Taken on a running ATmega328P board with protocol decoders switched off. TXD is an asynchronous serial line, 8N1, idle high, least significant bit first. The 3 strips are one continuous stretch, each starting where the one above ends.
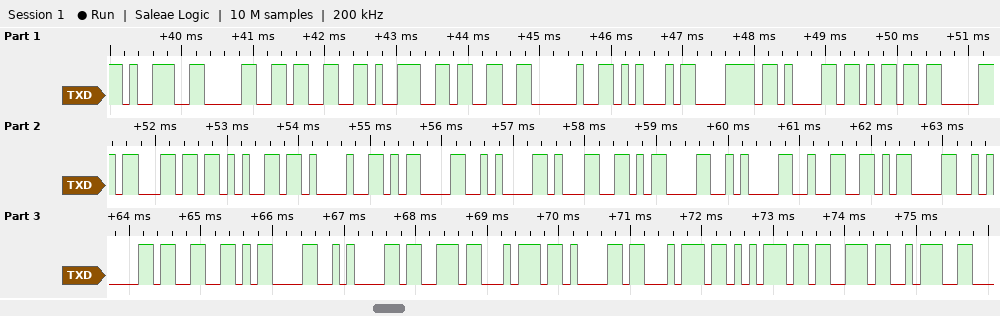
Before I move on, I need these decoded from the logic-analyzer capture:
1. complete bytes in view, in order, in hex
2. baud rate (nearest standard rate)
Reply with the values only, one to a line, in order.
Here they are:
39 30 33 39 33 20 45 78 61 6D 70 6C 65 21 0D 0A 31 0D 0A 32 0D 0A 33 0D 0A 73 74 61 74 75 73 3A
9600 baud
